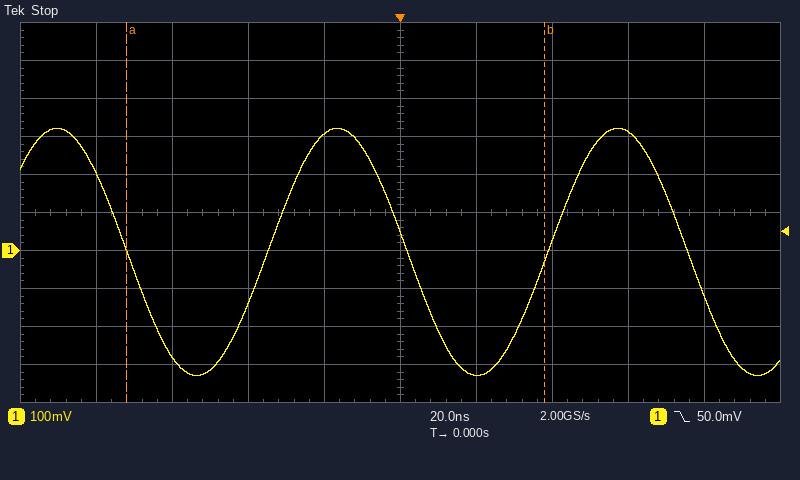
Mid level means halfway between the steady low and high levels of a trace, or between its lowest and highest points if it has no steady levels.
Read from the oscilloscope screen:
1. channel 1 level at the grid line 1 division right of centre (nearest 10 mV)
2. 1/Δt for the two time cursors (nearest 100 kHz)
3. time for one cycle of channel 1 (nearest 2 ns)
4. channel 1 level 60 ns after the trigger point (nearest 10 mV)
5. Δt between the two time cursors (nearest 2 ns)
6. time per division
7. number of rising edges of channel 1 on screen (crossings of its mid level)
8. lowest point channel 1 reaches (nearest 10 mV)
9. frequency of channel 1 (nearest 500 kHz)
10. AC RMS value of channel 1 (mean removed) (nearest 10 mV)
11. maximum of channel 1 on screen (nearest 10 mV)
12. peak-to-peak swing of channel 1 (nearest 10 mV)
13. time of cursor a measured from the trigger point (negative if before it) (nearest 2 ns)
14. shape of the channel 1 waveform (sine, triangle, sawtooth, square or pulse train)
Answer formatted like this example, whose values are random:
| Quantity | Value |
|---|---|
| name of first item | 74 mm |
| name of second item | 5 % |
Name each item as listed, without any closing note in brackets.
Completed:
| Quantity | Value |
|---|---|
| channel 1 level at the grid line 1 division right of centre | -330 mV |
| 1/Δt for the two time cursors | 9.1 MHz |
| time for one cycle of channel 1 | 74 ns |
| channel 1 level 60 ns after the trigger point | 310 mV |
| Δt between the two time cursors | 110 ns |
| time per division | 20 ns |
| number of rising edges of channel 1 on screen | 2 |
| lowest point channel 1 reaches | -330 mV |
| frequency of channel 1 | 13.5 MHz |
| AC RMS value of channel 1 (mean removed) | 230 mV |
| maximum of channel 1 on screen | 320 mV |
| peak-to-peak swing of channel 1 | 650 mV |
| time of cursor a measured from the trigger point (negative if before it) | -72 ns |
| shape of the channel 1 waveform | sine |
